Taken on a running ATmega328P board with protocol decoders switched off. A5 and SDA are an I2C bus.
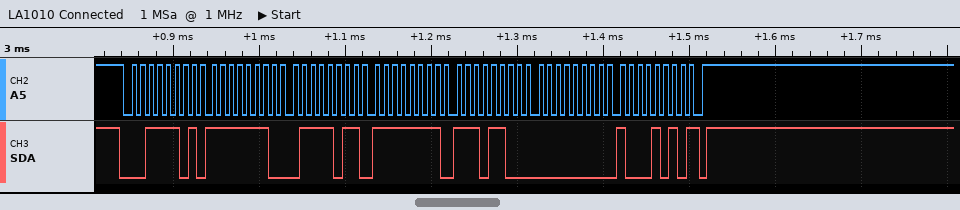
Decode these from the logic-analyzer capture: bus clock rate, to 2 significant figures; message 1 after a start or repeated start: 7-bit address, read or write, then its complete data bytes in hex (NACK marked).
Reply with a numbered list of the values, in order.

1. 100 kHz
2. 0x1E read: FE 7B FF EC 00 8A NACK
